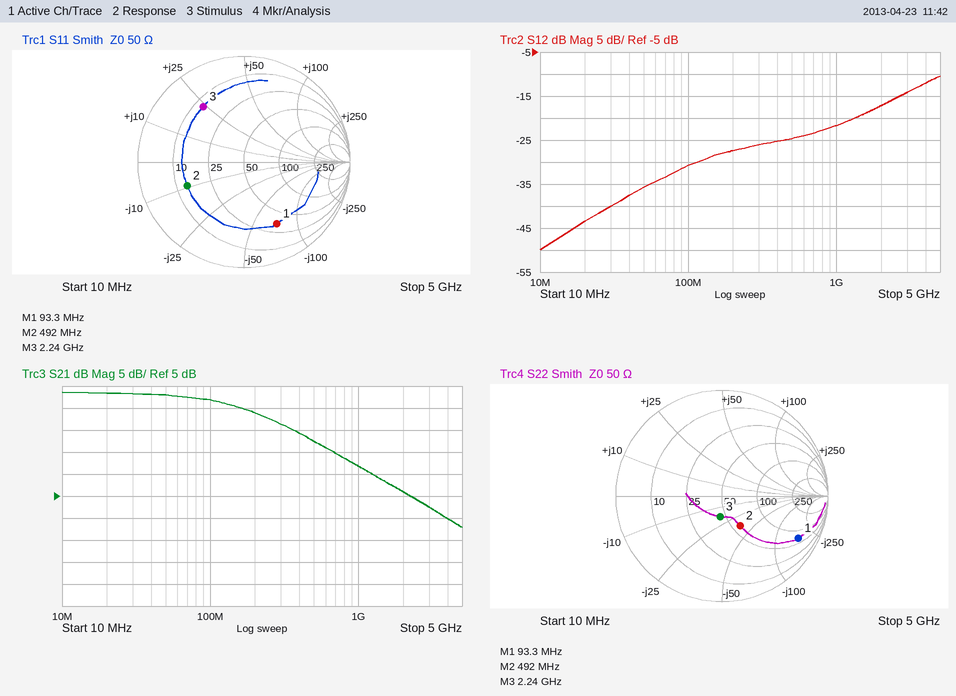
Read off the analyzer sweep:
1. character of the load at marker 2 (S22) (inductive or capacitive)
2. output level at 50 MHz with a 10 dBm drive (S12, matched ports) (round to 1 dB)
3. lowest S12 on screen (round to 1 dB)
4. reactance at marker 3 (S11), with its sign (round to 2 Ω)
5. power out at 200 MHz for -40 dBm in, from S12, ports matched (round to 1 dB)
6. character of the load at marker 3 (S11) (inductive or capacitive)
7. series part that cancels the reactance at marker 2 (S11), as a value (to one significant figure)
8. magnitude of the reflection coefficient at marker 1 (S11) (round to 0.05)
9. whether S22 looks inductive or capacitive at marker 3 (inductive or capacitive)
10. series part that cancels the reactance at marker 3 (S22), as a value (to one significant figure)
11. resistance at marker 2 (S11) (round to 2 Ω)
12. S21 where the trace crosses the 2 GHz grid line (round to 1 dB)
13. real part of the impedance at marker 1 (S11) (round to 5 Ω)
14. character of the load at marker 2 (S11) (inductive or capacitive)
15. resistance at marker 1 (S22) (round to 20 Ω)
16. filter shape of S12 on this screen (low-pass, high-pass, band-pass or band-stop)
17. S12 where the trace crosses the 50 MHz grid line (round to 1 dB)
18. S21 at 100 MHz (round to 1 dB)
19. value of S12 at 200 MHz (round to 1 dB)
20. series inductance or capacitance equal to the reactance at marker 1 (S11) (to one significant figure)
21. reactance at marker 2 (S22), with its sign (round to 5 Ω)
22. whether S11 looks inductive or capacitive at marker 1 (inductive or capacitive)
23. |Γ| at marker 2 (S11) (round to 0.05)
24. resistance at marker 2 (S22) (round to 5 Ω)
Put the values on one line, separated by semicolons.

capacitive; -26 dBm; -50 dB; +24 Ω; -67 dBm; inductive; 3 nH; 0.65; capacitive; 1 nH; 14 Ω; 6 dB; 35 Ω; capacitive; 60 Ω; high-pass; -36 dB; 27 dB; -27 dB; 20 pF; -35 Ω; capacitive; 0.60; 60 Ω
